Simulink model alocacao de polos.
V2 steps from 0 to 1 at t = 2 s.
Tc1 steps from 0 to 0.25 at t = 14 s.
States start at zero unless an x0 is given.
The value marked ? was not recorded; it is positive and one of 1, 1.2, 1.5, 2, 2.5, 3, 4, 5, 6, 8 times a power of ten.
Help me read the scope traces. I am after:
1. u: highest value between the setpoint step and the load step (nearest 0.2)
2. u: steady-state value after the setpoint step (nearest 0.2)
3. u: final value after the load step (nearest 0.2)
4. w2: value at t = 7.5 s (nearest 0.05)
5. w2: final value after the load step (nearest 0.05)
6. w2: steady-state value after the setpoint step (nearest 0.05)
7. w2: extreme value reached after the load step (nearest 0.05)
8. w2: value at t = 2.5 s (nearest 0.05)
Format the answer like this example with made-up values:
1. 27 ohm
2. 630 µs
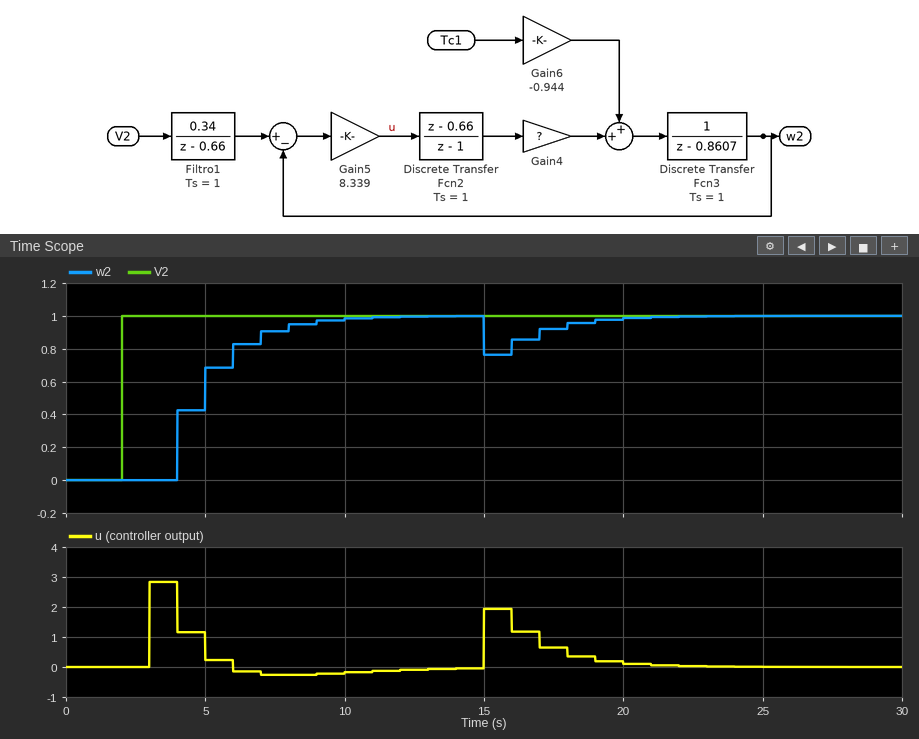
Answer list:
1. 2.8
2. 0.0
3. 0.0
4. 0.90
5. 1.00
6. 1.00
7. 0.75
8. 0.00
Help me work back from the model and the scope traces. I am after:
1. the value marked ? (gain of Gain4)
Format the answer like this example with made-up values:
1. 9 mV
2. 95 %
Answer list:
1. 0.15
